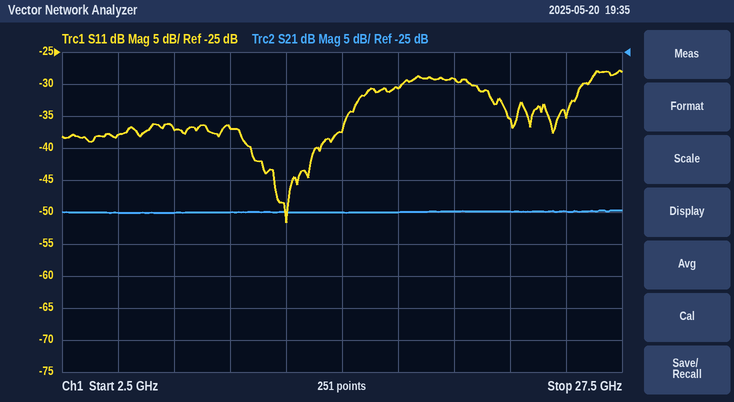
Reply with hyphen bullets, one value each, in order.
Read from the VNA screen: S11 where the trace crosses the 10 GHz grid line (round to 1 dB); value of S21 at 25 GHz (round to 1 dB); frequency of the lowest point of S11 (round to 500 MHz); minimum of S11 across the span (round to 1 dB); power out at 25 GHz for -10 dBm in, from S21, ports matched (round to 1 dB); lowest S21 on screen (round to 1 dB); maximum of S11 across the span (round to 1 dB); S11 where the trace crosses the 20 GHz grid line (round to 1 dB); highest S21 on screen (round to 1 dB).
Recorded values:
- -37 dB
- -50 dB
- 12.5 GHz
- -52 dB
- -60 dBm
- -50 dB
- -28 dB
- -29 dB
- -50 dB
